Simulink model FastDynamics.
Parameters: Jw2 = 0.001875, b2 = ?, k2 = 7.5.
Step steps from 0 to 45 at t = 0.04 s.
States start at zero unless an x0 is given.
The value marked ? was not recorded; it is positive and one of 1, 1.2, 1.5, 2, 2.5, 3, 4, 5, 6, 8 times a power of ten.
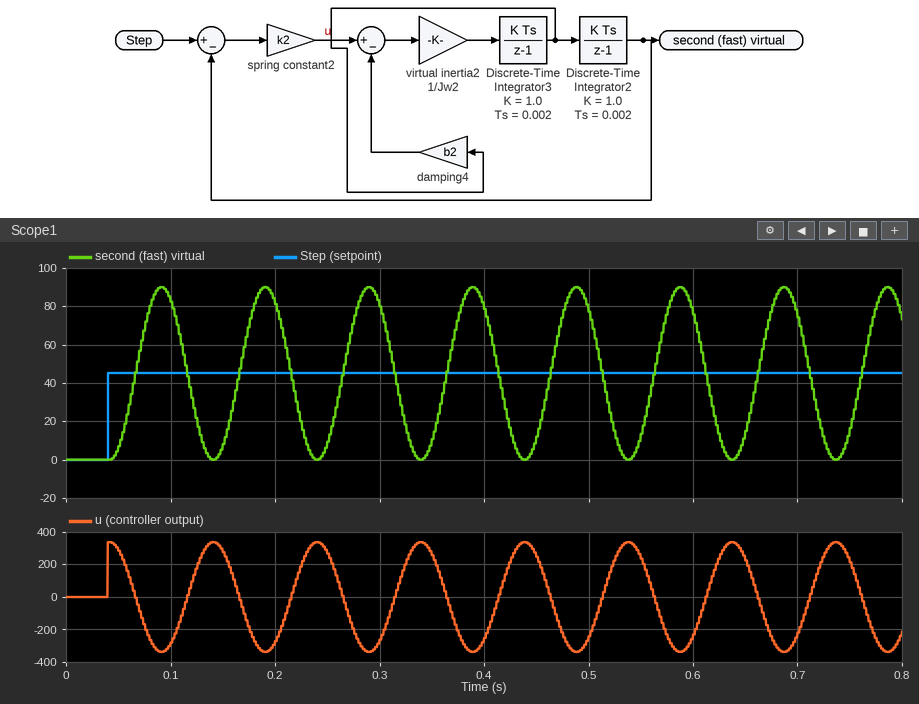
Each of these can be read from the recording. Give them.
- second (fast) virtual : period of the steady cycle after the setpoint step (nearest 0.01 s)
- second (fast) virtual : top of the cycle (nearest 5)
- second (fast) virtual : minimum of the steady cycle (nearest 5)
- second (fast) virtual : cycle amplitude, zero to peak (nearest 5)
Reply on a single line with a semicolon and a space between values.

0.10 s; 90; 0; 45
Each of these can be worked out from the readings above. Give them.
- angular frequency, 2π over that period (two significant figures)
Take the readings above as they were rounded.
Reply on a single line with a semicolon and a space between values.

63 rad/s
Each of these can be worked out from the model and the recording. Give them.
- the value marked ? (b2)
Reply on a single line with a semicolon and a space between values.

0.015
